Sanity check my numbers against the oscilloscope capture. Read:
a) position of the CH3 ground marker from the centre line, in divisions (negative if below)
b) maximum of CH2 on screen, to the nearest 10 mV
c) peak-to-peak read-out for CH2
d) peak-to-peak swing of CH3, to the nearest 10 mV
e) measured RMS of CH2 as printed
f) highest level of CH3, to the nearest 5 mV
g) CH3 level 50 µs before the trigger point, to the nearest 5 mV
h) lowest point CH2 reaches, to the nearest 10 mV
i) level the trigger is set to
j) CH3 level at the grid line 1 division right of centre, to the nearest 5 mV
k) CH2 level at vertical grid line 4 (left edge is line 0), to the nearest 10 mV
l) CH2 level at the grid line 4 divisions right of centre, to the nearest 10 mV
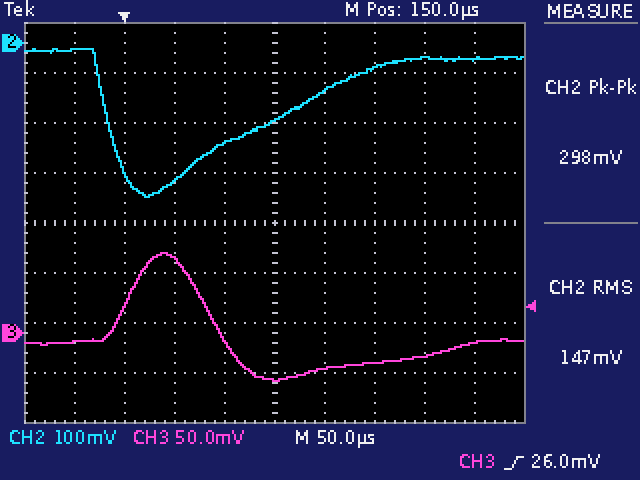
-2.2 div
-10 mV
298 mV
130 mV
147 mV
80 mV
-10 mV
-310 mV
26.0 mV
-35 mV
-200 mV
-30 mV
